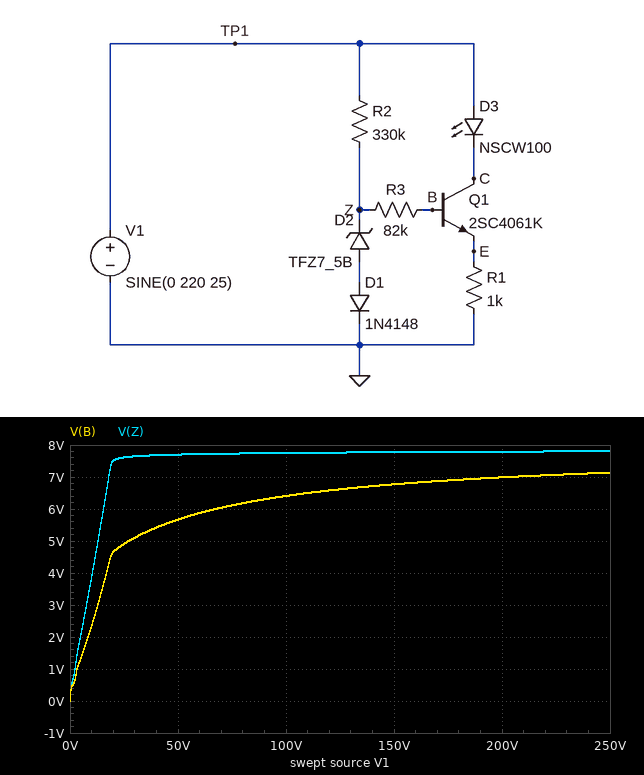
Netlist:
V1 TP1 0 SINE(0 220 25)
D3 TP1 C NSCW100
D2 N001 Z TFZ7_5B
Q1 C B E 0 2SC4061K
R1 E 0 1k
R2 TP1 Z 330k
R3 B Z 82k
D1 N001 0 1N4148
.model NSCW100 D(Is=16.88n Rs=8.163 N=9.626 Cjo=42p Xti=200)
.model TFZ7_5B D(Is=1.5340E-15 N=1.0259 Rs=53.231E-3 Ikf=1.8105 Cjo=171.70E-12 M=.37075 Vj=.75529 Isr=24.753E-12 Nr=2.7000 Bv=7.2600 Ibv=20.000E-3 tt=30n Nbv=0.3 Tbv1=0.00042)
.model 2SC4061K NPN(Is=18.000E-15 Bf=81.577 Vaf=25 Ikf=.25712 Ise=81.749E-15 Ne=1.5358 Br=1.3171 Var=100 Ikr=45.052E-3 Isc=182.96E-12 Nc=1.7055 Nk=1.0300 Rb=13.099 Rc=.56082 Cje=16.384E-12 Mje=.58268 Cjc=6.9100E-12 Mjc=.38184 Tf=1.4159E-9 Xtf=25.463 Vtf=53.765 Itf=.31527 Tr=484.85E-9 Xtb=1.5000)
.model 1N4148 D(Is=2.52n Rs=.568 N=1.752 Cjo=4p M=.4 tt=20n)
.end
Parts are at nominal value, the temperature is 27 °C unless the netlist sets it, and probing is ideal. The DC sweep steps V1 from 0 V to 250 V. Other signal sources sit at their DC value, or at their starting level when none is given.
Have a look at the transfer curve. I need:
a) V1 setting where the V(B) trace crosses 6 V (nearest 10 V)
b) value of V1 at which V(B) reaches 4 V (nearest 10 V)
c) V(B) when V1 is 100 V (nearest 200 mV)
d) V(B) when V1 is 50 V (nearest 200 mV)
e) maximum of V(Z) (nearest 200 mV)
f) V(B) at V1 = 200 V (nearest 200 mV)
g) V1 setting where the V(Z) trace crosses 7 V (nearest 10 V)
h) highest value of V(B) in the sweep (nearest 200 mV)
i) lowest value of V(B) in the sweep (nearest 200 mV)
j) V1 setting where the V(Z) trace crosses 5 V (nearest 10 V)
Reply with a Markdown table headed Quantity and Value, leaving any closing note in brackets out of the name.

| Quantity | Value |
|---|---|
| V1 setting where the V(B) trace crosses 6 V | 70 V |
| value of V1 at which V(B) reaches 4 V | 20 V |
| V(B) when V1 is 100 V | 6.4 V |
| V(B) when V1 is 50 V | 5.6 V |
| maximum of V(Z) | 7.8 V |
| V(B) at V1 = 200 V | 7.0 V |
| V1 setting where the V(Z) trace crosses 7 V | 20 V |
| highest value of V(B) in the sweep | 7.2 V |
| lowest value of V(B) in the sweep | 0 V |
| V1 setting where the V(Z) trace crosses 5 V | 10 V |
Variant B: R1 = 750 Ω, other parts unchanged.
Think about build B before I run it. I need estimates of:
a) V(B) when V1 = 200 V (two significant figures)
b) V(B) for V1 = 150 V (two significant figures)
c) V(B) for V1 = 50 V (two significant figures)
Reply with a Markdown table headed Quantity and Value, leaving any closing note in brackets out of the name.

| Quantity | Value |
|---|---|
| V(B) when V1 = 200 V | 6.8 V |
| V(B) for V1 = 150 V | 6.5 V |
| V(B) for V1 = 50 V | 5.2 V |
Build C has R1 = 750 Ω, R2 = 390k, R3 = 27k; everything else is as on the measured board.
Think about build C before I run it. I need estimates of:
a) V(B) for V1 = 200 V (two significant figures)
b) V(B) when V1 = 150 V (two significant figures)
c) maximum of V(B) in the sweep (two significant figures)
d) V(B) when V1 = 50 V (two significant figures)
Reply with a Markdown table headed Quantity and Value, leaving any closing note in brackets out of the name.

| Quantity | Value |
|---|---|
| V(B) for V1 = 200 V | 7.4 V |
| V(B) when V1 = 150 V | 7.3 V |
| maximum of V(B) in the sweep | 7.5 V |
| V(B) when V1 = 50 V | 6.6 V |
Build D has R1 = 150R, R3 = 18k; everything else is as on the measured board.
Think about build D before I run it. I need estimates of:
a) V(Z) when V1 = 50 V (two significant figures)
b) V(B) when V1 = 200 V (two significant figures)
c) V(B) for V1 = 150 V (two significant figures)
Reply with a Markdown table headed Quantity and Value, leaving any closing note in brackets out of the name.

| Quantity | Value |
|---|---|
| V(Z) when V1 = 50 V | 6.9 V |
| V(B) when V1 = 200 V | 6.7 V |
| V(B) for V1 = 150 V | 6.4 V |
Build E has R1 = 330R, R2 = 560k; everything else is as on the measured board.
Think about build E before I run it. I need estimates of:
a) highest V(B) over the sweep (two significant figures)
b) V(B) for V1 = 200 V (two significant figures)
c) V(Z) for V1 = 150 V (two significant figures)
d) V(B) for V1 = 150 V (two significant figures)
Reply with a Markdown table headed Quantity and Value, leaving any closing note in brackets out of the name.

| Quantity | Value |
|---|---|
| highest V(B) over the sweep | 6.1 V |
| V(B) for V1 = 200 V | 5.8 V |
| V(Z) for V1 = 150 V | 7.7 V |
| V(B) for V1 = 150 V | 5.4 V |
